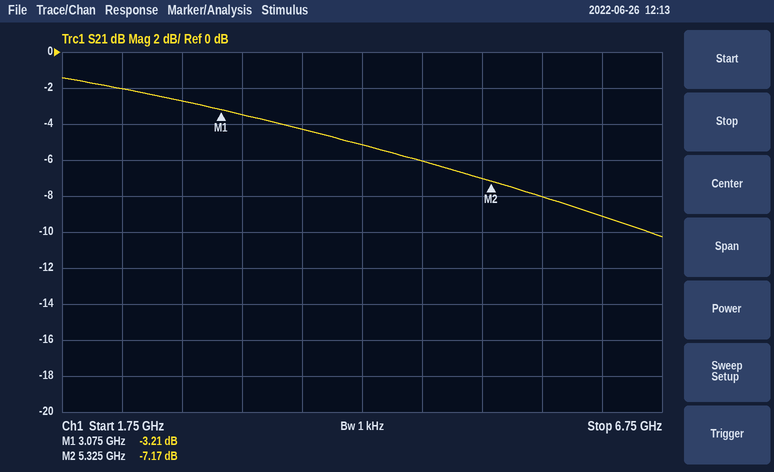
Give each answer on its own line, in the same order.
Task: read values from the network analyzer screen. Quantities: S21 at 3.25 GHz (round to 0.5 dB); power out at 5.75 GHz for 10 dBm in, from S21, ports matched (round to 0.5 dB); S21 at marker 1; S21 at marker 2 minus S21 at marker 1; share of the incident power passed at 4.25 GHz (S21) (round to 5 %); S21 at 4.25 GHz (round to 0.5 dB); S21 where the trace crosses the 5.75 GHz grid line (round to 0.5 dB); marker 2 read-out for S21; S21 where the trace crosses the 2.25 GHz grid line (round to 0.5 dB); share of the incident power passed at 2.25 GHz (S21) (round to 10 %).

-3.5 dB
2.0 dBm
-3.21 dB
-3.96 dB
30 %
-5.0 dB
-8.0 dB
-7.17 dB
-2.0 dB
60 %
